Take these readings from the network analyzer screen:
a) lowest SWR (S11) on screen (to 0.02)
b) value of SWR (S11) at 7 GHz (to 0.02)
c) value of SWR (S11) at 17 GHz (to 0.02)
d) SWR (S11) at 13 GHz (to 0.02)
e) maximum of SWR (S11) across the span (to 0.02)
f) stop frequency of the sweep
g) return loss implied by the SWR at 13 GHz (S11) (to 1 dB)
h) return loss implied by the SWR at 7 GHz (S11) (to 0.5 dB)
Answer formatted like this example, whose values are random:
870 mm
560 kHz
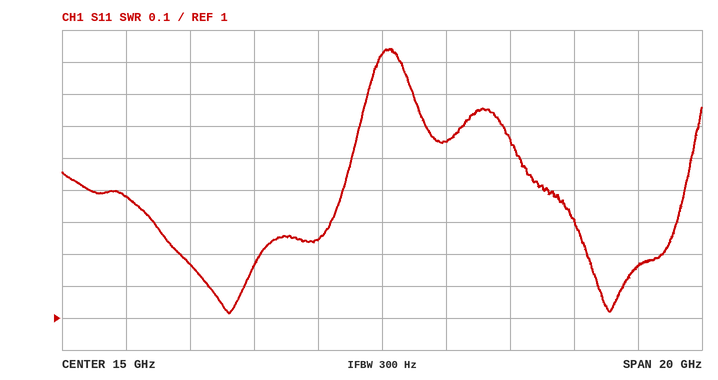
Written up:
1.02
1.38
1.56
1.24
1.84
25 GHz
19 dB
16.0 dB
